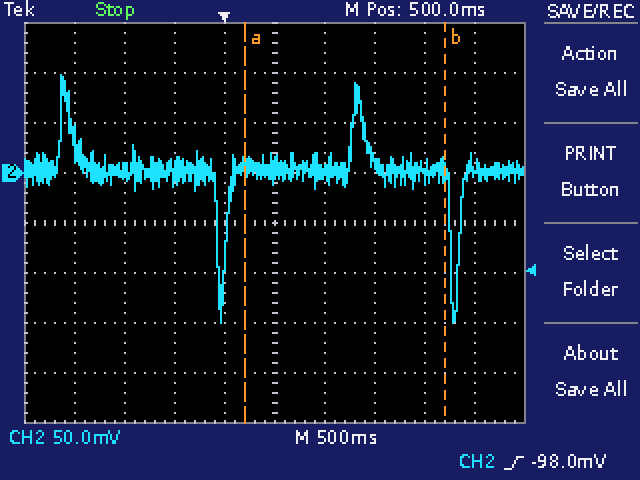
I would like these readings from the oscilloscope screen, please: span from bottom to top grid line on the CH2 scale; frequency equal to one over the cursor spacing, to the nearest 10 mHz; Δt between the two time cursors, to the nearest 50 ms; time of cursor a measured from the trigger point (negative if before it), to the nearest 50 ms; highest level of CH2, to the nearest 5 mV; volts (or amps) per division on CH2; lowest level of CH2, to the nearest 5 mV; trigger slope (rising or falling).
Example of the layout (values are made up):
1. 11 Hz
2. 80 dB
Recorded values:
1. 400 mV
2. 500 mHz
3. 2.00 s
4. +200 ms
5. 100 mV
6. 50 mV
7. -150 mV
8. rising
